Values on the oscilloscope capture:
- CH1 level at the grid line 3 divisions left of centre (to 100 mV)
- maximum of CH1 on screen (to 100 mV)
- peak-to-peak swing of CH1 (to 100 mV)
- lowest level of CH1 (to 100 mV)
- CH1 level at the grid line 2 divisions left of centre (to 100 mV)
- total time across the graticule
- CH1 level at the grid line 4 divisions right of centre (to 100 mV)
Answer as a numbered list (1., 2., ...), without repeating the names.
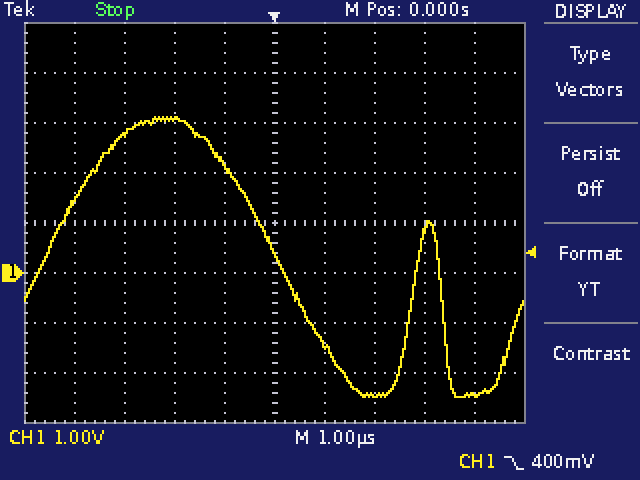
1. 2.8 V
2. 3.1 V
3. 5.6 V
4. -2.5 V
5. 3.1 V
6. 10 µs
7. -2.4 V
